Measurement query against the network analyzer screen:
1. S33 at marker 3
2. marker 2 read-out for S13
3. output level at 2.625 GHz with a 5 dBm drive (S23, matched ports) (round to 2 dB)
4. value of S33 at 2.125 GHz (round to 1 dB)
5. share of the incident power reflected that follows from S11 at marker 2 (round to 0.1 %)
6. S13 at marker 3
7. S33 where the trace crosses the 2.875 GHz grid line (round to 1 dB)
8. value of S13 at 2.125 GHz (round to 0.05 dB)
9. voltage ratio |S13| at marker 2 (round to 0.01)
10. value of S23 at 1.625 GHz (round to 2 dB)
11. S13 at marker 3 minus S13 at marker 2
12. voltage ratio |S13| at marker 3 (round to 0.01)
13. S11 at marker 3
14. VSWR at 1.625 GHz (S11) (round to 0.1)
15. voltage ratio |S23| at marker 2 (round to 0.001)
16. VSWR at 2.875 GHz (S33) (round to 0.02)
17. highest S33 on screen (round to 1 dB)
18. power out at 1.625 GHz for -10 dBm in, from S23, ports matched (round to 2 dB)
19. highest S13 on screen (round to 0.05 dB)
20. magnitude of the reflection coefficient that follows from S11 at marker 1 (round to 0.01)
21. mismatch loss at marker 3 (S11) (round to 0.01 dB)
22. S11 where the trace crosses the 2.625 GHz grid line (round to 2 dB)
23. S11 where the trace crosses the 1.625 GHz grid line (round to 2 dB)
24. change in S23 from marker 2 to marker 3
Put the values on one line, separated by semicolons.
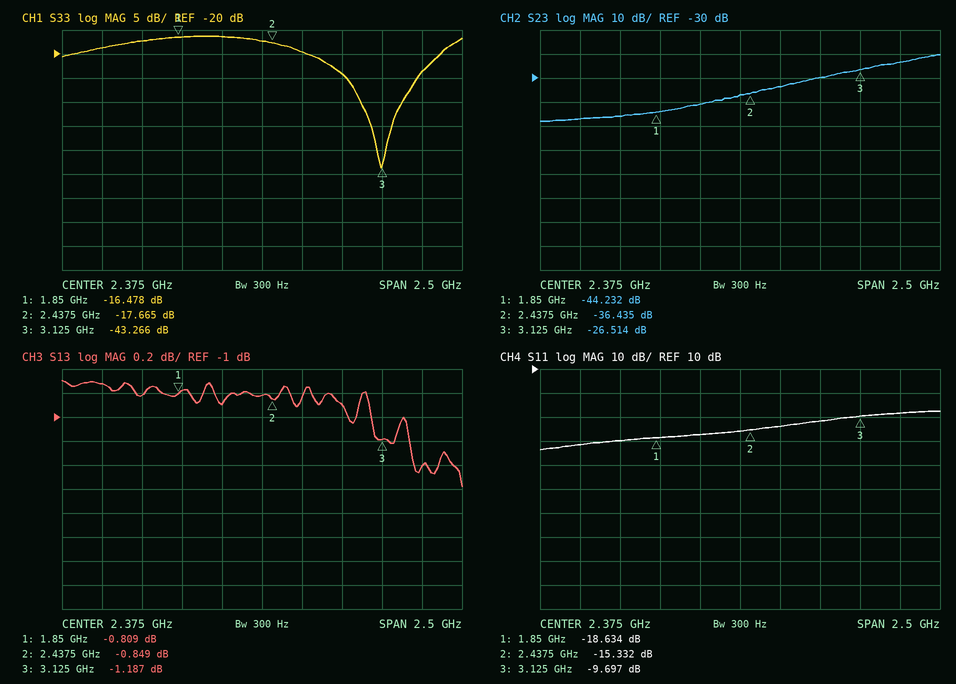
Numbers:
-43.266 dB; -0.849 dB; -28 dBm; -16 dB; 2.9 %; -1.187 dB; -24 dB; -0.90 dB; 0.91; -46 dB; -0.338 dB; 0.87; -9.697 dB; 1.2; 0.015; 1.14; -16 dB; -56 dBm; -0.70 dB; 0.12; 0.49 dB; -14 dB; -20 dB; 9.921 dB
